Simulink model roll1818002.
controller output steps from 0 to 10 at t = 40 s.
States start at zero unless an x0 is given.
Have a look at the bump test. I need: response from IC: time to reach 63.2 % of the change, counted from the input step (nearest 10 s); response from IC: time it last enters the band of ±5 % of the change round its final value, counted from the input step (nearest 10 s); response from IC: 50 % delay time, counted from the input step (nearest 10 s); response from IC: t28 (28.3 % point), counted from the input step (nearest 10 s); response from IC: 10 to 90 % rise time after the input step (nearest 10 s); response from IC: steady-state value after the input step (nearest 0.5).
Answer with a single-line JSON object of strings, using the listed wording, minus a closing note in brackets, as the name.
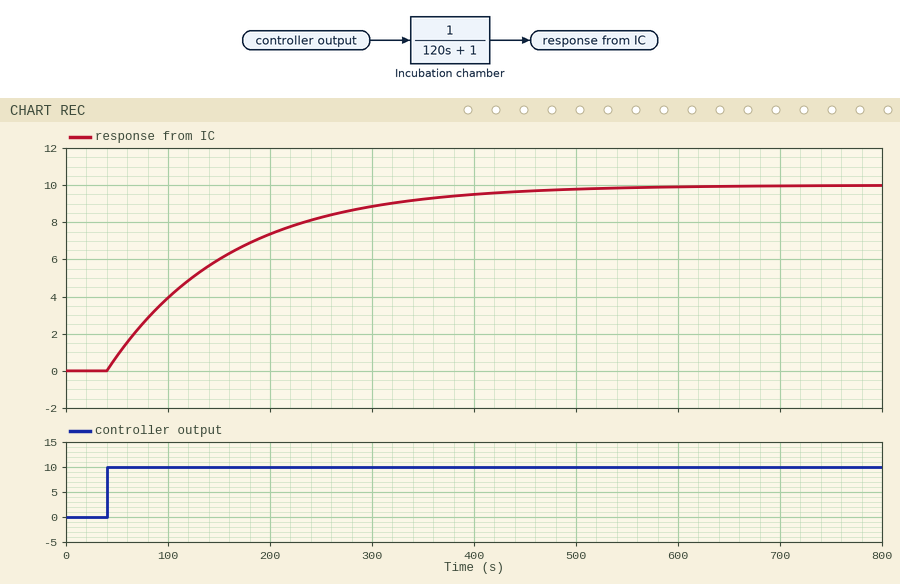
{"response from IC: time to reach 63.2 % of the change, counted from the input step": "120 s", "response from IC: time it last enters the band of ±5 % of the change round its final value, counted from the input step": "360 s", "response from IC: 50 % delay time, counted from the input step": "80 s", "response from IC: t28 (28.3 % point), counted from the input step": "40 s", "response from IC: 10 to 90 % rise time after the input step": "260 s", "response from IC: steady-state value after the input step": "10.0"}
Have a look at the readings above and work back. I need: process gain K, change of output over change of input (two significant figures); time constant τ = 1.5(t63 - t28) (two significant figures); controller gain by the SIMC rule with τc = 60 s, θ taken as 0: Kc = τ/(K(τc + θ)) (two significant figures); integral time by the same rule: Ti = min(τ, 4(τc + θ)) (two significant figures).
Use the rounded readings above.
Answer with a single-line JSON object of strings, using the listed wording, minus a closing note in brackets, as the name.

{"process gain K, change of output over change of input": "1.0", "time constant τ = 1.5(t63 - t28)": "120 s", "controller gain by the SIMC rule with τc = 60 s, θ taken as 0: Kc = τ/(K(τc + θ))": "2.0", "integral time by the same rule: Ti = min(τ, 4(τc + θ))": "120 s"}
